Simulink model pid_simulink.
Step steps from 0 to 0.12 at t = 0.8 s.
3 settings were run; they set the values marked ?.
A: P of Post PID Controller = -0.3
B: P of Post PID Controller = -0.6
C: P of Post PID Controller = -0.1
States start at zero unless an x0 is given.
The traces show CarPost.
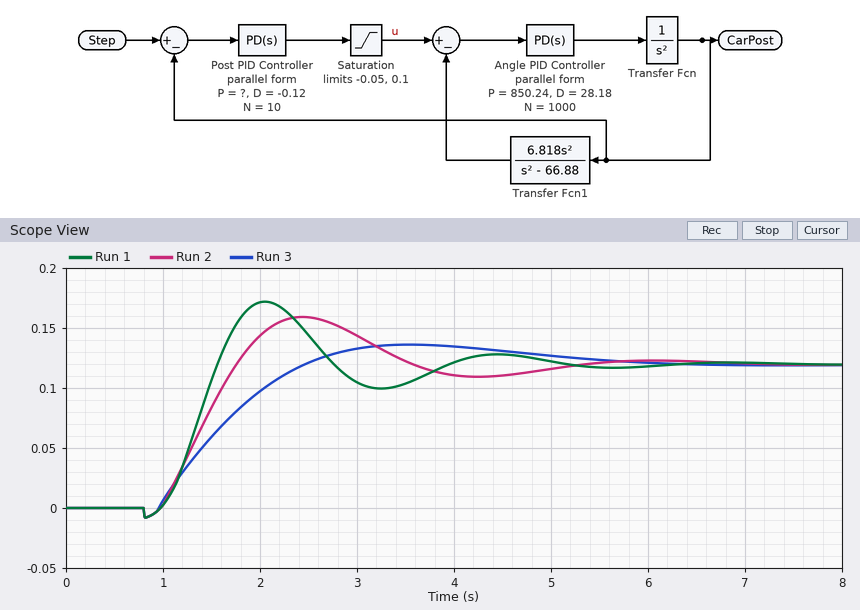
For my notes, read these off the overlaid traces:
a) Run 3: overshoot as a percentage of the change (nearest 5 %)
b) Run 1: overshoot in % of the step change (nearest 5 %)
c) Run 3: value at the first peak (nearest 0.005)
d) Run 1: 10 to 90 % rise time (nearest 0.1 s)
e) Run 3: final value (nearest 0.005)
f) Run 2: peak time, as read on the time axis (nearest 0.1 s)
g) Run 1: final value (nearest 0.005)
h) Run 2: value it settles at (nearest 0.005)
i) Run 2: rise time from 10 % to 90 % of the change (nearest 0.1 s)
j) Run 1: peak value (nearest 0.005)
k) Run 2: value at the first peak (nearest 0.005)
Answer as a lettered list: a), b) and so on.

a) 15 %
b) 45 %
c) 0.135
d) 0.4 s
e) 0.120
f) 2.4 s
g) 0.120
h) 0.120
i) 0.6 s
j) 0.170
k) 0.160
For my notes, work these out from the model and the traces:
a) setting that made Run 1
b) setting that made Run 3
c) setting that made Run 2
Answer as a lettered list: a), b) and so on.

a) B
b) C
c) A
